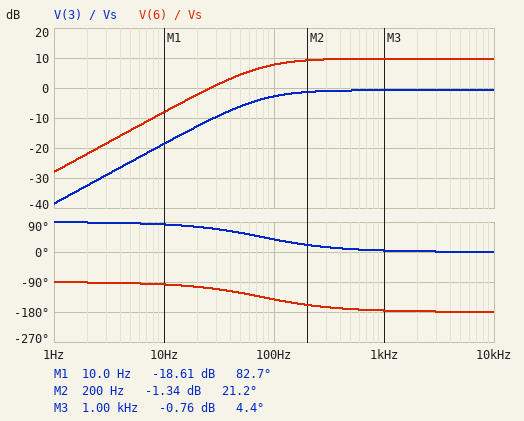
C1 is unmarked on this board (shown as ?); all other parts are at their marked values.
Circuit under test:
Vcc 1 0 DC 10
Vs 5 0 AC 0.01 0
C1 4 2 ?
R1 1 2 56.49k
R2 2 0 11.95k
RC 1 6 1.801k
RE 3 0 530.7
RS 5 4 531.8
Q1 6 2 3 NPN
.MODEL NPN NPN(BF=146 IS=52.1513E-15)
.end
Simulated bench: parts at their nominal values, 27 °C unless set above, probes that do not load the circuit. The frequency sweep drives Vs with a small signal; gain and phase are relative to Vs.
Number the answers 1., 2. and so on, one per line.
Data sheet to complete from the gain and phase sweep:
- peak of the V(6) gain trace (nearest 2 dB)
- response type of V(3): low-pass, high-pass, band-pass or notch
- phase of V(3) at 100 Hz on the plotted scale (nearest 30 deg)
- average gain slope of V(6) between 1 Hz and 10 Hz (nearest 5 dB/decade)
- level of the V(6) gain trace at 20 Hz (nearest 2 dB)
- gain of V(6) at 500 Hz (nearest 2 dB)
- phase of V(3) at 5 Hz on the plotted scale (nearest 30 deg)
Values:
1. 10 dB
2. high-pass
3. 30 deg
4. 20 dB/decade
5. -2 dB
6. 10 dB
7. 90 deg
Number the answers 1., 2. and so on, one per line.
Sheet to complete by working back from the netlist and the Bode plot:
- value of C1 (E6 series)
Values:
1. 220 nF
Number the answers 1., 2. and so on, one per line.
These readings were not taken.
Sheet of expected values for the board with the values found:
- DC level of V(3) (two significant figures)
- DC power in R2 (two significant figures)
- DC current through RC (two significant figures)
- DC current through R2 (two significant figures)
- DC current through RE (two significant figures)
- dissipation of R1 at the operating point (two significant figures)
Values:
1. 990 mV
2. 220 µW
3. 1.9 mA
4. 140 µA
5. 1.9 mA
6. 1.2 mW
